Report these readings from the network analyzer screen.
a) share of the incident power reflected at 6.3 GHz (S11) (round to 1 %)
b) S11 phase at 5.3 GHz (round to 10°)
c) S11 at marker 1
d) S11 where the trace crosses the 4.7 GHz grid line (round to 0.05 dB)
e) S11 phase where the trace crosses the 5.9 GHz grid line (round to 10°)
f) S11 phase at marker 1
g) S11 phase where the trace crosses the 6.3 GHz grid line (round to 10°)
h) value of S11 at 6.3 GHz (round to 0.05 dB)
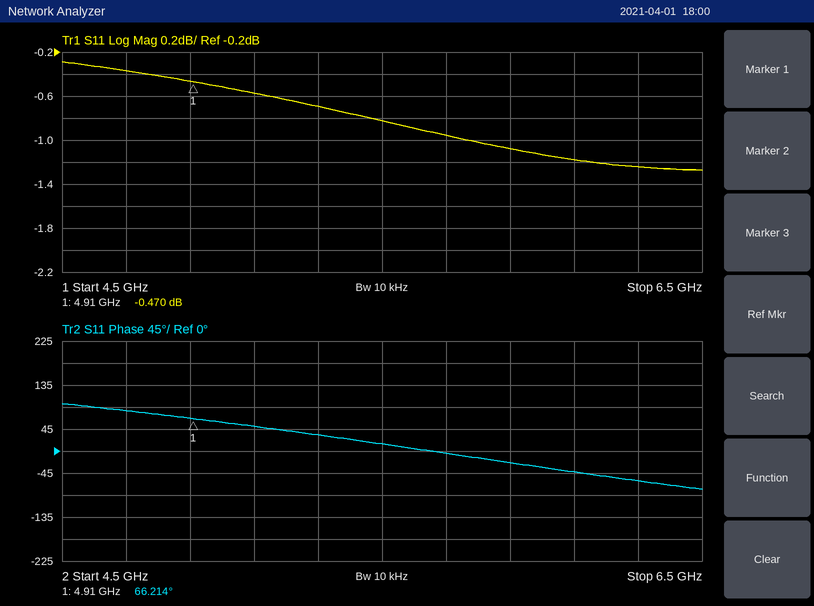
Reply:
75 %
30°
-0.470 dB
-0.35 dB
-20°
66.214°
-60°
-1.25 dB
